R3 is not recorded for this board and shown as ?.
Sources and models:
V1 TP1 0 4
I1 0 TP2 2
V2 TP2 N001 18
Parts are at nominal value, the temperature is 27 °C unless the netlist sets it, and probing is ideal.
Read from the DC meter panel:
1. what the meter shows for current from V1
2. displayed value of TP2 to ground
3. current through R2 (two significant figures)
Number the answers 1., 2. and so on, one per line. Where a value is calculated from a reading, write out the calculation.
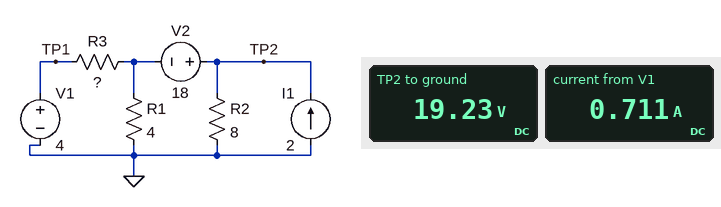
1. 0.711 A
2. 19.23 V
3. (19.23 V) / 8 Ω = 2.4 A
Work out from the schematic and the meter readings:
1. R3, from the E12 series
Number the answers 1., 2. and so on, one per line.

1. 3.9 Ω
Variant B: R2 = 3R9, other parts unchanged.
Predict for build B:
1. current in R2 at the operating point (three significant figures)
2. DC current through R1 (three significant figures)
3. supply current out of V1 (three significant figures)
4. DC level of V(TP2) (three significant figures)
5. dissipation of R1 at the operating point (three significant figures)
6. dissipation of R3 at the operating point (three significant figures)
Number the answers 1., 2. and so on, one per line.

1. 4.08 A
2. 521 mA
3. 1.56 A
4. 15.9 V
5. 1.09 W
6. 9.49 W
